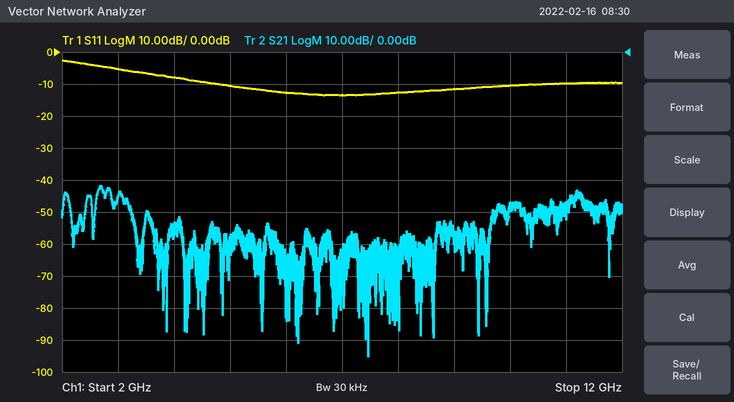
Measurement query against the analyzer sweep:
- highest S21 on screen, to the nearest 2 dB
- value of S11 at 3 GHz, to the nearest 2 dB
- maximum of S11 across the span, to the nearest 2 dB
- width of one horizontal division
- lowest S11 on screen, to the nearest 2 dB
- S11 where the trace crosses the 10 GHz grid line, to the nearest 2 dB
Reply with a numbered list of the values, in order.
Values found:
1. -42 dB
2. -6 dB
3. -2 dB
4. 1 GHz
5. -14 dB
6. -10 dB
